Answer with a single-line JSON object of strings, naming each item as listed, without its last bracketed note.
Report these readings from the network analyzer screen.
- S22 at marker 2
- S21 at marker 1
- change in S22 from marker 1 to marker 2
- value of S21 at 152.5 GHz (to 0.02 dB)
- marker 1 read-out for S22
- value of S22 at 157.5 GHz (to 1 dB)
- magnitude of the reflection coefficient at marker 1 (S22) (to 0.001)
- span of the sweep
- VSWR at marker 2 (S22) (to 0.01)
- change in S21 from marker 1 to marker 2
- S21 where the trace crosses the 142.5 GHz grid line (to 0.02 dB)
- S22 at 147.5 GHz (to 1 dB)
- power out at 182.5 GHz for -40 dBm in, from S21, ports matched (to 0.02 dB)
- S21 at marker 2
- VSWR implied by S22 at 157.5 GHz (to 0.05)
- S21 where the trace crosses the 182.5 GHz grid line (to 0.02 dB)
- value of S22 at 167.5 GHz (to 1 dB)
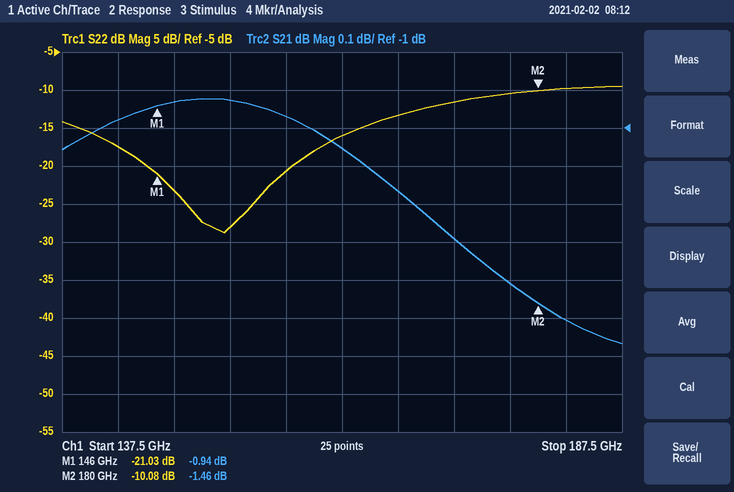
{"S22 at marker 2": "-10.08 dB", "S21 at marker 1": "-0.94 dB", "change in S22 from marker 1 to marker 2": "10.95 dB", "value of S21 at 152.5 GHz": "-0.92 dB", "marker 1 read-out for S22": "-21.03 dB", "value of S22 at 157.5 GHz": "-21 dB", "magnitude of the reflection coefficient at marker 1 (S22)": "0.089", "span of the sweep": "50 GHz", "VSWR at marker 2 (S22)": "1.91", "change in S21 from marker 1 to marker 2": "-0.52 dB", "S21 where the trace crosses the 142.5 GHz grid line": "-0.98 dB", "S22 at 147.5 GHz": "-23 dB", "power out at 182.5 GHz for -40 dBm in, from S21, ports matched": "-41.50 dBm", "S21 at marker 2": "-1.46 dB", "VSWR implied by S22 at 157.5 GHz": "1.20", "S21 where the trace crosses the 182.5 GHz grid line": "-1.50 dB", "value of S22 at 167.5 GHz": "-13 dB"}
